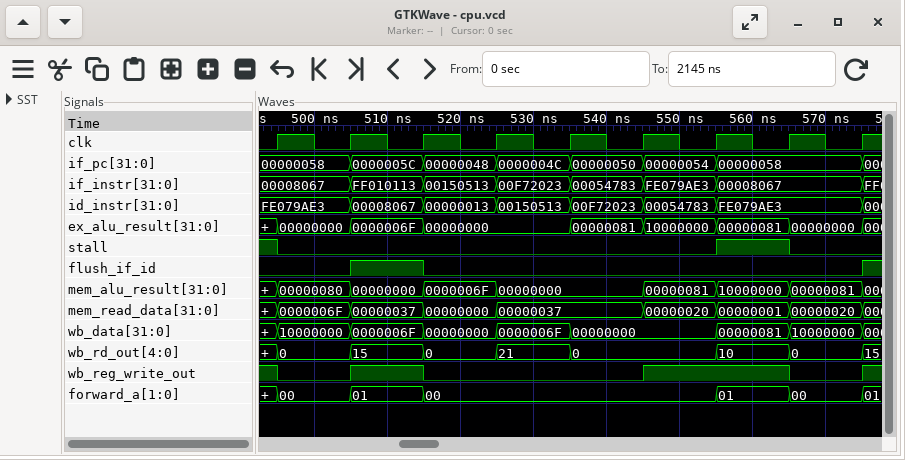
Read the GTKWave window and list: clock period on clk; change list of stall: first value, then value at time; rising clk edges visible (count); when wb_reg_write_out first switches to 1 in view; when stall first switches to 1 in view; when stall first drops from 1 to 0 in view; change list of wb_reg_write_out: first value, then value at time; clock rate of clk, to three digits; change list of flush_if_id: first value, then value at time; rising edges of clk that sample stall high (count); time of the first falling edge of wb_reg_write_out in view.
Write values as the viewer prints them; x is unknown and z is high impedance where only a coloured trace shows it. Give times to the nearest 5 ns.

10 ns
1, 0 at 495 ns, 1 at 555 ns, 0 at 565 ns
9
505 ns
555 ns
495 ns
1, 0 at 495 ns, 1 at 505 ns, 0 at 515 ns, 1 at 545 ns, 0 at 565 ns, 1 at 575 ns
100 MHz
0, 1 at 505 ns, 0 at 515 ns, 1 at 575 ns
2
495 ns
